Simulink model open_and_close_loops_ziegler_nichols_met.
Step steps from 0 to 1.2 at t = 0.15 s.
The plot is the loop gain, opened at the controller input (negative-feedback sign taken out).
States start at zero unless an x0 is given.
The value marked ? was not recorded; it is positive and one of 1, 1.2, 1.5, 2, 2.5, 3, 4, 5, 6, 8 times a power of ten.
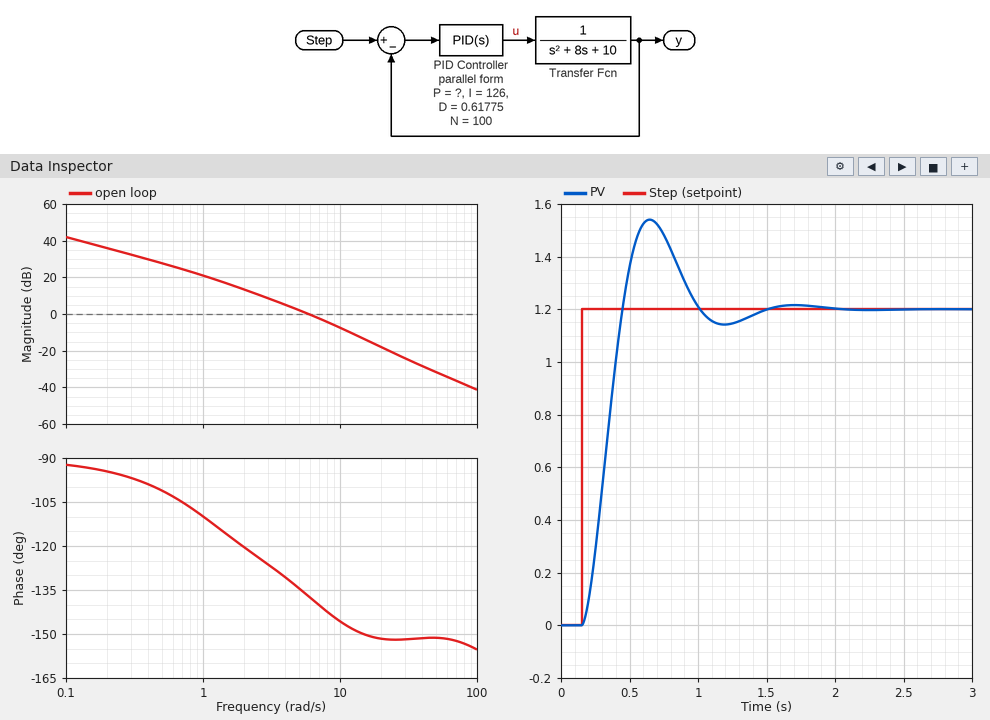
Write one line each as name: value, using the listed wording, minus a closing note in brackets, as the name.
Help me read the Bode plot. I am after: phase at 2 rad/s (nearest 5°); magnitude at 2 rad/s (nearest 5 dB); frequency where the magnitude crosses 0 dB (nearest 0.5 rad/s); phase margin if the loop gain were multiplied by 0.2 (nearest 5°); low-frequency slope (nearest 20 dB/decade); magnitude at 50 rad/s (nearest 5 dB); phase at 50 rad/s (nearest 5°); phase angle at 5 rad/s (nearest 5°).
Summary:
phase at 2 rad/s: -120°
magnitude at 2 rad/s: 15 dB
frequency where the magnitude crosses 0 dB: 6.0 rad/s
phase margin if the loop gain were multiplied by 0.2: 60°
low-frequency slope: -20 dB/decade
magnitude at 50 rad/s: -30 dB
phase at 50 rad/s: -150°
phase angle at 5 rad/s: -135°
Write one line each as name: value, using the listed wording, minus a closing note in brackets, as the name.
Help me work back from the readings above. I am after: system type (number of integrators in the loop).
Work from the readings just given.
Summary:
system type: 1
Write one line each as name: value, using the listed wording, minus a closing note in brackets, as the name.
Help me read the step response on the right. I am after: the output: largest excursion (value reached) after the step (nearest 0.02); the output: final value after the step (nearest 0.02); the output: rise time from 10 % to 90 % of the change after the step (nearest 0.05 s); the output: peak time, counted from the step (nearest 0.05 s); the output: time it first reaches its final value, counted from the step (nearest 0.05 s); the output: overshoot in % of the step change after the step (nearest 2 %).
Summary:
the output: largest excursion (value reached) after the step: 1.54
the output: final value after the step: 1.20
the output: rise time from 10 % to 90 % of the change after the step: 0.20 s
the output: peak time, counted from the step: 0.50 s
the output: time it first reaches its final value, counted from the step: 0.30 s
the output: overshoot in % of the step change after the step: 28 %
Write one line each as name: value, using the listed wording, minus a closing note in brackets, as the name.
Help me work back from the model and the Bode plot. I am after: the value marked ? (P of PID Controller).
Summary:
the value marked ?: 50
